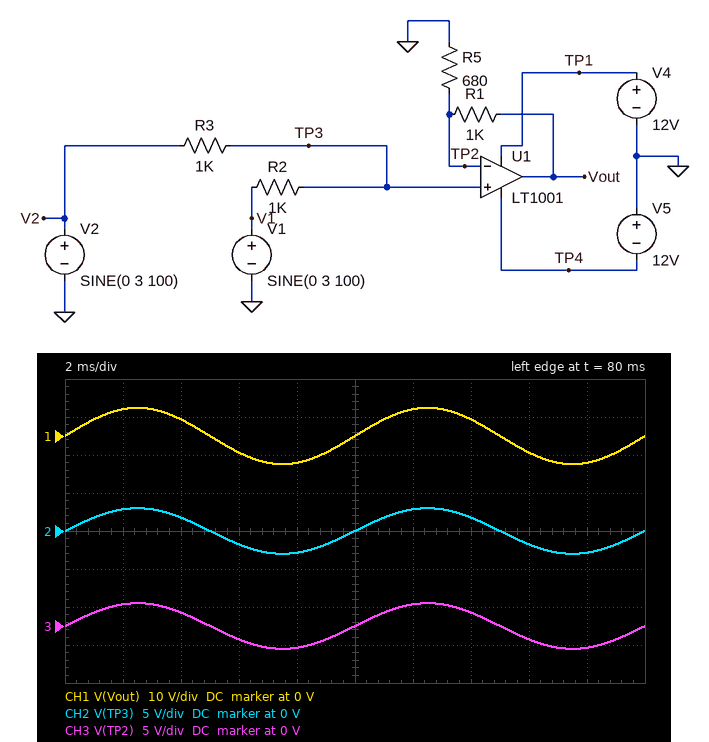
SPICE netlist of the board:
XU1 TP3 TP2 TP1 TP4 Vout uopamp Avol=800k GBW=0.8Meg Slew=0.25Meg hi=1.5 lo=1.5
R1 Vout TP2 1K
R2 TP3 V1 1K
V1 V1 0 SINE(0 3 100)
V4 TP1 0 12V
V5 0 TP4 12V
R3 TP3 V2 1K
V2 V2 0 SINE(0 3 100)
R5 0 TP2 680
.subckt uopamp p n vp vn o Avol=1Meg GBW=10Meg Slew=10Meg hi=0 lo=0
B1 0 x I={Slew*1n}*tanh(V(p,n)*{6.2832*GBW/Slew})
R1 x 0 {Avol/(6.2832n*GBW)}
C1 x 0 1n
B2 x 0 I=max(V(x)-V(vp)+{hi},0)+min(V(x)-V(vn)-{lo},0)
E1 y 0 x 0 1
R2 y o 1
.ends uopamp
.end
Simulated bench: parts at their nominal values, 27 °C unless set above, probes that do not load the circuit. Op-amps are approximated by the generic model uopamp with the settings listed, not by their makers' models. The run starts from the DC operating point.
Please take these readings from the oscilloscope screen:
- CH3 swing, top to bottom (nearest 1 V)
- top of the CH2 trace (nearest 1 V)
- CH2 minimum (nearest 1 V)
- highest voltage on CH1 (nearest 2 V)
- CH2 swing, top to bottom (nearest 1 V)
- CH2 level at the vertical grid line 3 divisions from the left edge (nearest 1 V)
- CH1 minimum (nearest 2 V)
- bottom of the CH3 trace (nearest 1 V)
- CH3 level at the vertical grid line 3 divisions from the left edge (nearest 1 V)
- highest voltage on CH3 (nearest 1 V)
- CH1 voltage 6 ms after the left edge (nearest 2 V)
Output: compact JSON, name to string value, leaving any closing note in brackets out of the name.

{"CH3 swing, top to bottom": "6 V", "top of the CH2 trace": "3 V", "CH2 minimum": "-3 V", "highest voltage on CH1": "8 V", "CH2 swing, top to bottom": "6 V", "CH2 level at the vertical grid line 3 divisions from the left edge": "-2 V", "CH1 minimum": "-8 V", "bottom of the CH3 trace": "-3 V", "CH3 level at the vertical grid line 3 divisions from the left edge": "-2 V", "highest voltage on CH3": "3 V", "CH1 voltage 6 ms after the left edge": "-4 V"}
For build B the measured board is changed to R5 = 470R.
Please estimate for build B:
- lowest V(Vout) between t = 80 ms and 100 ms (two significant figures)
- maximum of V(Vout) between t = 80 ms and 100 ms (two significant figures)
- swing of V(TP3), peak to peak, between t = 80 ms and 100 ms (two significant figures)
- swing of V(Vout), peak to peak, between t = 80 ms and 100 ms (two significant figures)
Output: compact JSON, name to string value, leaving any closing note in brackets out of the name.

{"lowest V(Vout) between t = 80 ms and 100 ms": "-9.4 V", "maximum of V(Vout) between t = 80 ms and 100 ms": "9.4 V", "swing of V(TP3), peak to peak, between t = 80 ms and 100 ms": "6.0 V", "swing of V(Vout), peak to peak, between t = 80 ms and 100 ms": "19 V"}
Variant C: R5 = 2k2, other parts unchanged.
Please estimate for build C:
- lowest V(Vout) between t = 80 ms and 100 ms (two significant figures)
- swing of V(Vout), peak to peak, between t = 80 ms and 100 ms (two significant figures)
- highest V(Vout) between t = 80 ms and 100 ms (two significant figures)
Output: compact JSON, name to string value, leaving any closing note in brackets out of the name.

{"lowest V(Vout) between t = 80 ms and 100 ms": "-4.4 V", "swing of V(Vout), peak to peak, between t = 80 ms and 100 ms": "8.7 V", "highest V(Vout) between t = 80 ms and 100 ms": "4.4 V"}
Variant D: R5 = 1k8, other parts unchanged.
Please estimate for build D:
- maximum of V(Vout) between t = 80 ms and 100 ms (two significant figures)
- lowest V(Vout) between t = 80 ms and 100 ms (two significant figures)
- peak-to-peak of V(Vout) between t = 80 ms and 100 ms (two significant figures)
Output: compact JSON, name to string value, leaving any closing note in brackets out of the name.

{"maximum of V(Vout) between t = 80 ms and 100 ms": "4.7 V", "lowest V(Vout) between t = 80 ms and 100 ms": "-4.7 V", "peak-to-peak of V(Vout) between t = 80 ms and 100 ms": "9.3 V"}
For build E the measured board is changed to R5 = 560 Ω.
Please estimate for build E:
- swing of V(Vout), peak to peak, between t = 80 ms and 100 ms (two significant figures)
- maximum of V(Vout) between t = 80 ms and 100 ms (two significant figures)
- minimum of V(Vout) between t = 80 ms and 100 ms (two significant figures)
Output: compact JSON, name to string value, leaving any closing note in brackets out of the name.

{"swing of V(Vout), peak to peak, between t = 80 ms and 100 ms": "17 V", "maximum of V(Vout) between t = 80 ms and 100 ms": "8.4 V", "minimum of V(Vout) between t = 80 ms and 100 ms": "-8.4 V"}
